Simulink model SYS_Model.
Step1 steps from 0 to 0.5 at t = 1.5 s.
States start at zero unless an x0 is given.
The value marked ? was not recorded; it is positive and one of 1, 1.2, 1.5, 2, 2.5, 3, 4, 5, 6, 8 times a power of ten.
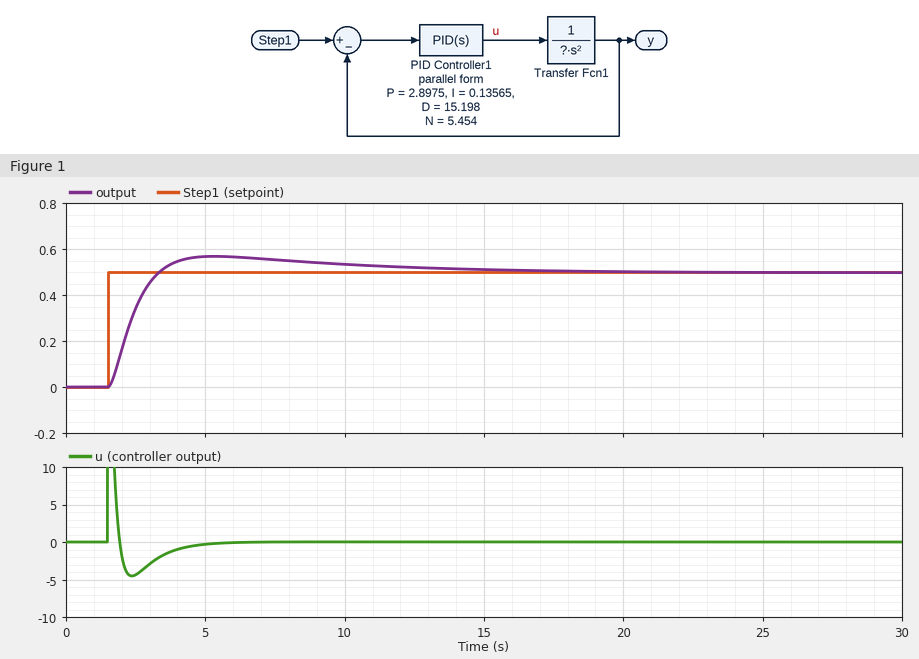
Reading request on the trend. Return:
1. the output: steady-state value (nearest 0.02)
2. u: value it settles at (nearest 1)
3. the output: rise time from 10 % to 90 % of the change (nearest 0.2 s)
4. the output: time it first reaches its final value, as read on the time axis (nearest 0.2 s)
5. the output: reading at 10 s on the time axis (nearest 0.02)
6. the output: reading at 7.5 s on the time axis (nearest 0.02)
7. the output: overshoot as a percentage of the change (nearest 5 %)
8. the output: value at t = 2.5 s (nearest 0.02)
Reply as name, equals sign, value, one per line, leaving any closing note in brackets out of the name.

the output: steady-state value = 0.50
u: value it settles at = 0
the output: rise time from 10 % to 90 % of the change = 1.2 s
the output: time it first reaches its final value, as read on the time axis = 3.4 s
the output: reading at 10 s on the time axis = 0.54
the output: reading at 7.5 s on the time axis = 0.56
the output: overshoot as a percentage of the change = 15 %
the output: value at t = 2.5 s = 0.34
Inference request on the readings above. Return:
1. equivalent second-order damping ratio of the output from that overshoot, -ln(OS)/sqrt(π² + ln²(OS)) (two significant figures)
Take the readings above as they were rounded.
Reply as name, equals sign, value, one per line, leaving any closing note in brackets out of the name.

equivalent second-order damping ratio of the output from that overshoot, -ln(OS)/sqrt(π² + ln²(OS)) = 0.52
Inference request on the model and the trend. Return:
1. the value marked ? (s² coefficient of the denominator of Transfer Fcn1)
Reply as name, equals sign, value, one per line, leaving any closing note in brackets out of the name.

the value marked ? = 15
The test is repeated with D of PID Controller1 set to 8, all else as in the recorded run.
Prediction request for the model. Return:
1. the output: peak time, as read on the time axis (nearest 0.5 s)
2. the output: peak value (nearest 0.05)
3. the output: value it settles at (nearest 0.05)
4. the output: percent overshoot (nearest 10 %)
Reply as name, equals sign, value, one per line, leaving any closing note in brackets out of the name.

the output: peak time, as read on the time axis = 6.5 s
the output: peak value = 0.65
the output: value it settles at = 0.50
the output: percent overshoot = 30 %
